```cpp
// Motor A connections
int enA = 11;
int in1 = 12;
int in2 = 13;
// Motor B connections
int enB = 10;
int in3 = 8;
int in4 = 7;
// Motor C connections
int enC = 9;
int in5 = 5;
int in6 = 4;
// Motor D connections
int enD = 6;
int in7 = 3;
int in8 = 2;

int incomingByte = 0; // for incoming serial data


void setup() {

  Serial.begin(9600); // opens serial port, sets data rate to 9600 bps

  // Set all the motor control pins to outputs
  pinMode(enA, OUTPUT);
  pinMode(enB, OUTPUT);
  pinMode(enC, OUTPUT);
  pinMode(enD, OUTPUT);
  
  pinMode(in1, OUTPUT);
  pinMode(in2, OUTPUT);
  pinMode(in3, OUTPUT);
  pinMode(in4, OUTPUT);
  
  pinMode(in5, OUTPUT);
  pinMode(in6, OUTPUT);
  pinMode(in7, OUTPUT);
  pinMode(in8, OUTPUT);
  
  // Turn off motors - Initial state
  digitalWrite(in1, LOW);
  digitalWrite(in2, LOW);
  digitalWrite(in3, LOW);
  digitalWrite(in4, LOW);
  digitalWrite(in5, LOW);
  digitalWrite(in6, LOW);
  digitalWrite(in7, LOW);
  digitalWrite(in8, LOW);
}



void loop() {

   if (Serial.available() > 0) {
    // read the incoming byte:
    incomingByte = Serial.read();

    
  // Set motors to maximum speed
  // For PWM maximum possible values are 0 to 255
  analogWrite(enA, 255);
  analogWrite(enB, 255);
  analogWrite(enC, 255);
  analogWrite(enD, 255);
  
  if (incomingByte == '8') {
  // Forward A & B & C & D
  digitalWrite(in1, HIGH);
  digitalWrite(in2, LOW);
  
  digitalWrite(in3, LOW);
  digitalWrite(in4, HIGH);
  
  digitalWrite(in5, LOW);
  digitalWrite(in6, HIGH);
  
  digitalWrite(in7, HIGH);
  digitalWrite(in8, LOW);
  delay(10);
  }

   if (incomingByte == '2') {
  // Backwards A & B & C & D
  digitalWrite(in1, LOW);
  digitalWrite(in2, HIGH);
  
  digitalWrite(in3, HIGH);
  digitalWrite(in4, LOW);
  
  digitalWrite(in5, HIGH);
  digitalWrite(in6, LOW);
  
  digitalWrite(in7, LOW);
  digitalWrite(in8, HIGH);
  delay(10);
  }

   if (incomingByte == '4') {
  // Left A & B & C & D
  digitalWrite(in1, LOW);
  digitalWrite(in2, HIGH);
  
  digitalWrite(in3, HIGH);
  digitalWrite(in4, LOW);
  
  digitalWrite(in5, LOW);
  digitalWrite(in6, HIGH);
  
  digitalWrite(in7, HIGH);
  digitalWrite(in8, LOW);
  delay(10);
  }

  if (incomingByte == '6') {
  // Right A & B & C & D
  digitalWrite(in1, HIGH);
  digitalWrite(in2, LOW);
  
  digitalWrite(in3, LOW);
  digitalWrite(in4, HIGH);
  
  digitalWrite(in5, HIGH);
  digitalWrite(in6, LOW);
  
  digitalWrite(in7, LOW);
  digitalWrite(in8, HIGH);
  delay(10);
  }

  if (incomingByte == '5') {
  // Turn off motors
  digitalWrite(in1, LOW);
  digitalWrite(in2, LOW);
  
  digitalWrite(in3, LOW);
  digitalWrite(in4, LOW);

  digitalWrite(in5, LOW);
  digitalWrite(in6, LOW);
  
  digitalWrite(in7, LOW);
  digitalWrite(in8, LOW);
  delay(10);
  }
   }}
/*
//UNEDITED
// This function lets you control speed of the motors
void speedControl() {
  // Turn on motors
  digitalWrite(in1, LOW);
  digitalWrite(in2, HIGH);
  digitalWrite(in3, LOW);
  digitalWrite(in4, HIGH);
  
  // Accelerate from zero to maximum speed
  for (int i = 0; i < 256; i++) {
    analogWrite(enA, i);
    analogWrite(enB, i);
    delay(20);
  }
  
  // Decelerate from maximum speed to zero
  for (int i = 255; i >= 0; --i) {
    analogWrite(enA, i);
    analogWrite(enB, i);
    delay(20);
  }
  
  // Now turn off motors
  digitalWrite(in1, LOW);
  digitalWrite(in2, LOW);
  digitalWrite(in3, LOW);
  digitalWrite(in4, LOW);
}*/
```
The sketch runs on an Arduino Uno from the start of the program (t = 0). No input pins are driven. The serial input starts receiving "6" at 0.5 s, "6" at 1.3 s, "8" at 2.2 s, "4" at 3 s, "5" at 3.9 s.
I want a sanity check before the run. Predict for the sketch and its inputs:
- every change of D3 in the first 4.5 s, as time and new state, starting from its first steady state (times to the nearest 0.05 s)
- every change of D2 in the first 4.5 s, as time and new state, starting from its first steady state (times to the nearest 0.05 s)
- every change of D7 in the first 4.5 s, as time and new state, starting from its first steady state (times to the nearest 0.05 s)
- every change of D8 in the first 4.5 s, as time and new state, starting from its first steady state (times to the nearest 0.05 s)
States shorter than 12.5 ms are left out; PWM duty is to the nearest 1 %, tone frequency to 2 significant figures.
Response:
0 s low; 2.2 s high; 3.9 s low
0 s low; 0.5 s high; 2.2 s low
0 s low; 0.5 s high; 3 s low
0 s low; 3 s high; 3.9 s low
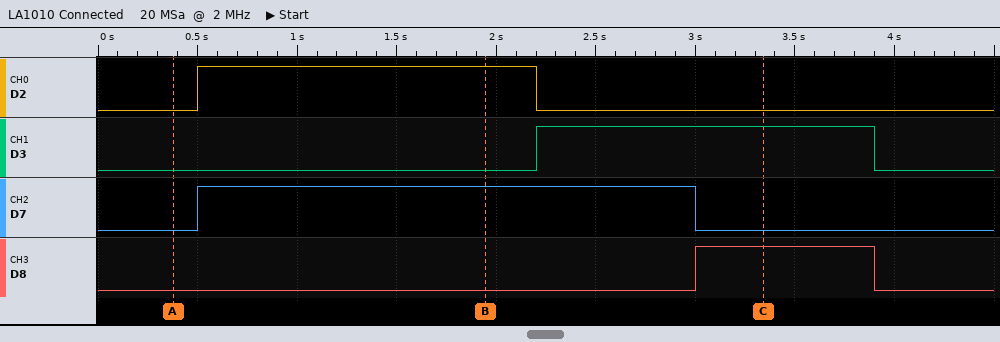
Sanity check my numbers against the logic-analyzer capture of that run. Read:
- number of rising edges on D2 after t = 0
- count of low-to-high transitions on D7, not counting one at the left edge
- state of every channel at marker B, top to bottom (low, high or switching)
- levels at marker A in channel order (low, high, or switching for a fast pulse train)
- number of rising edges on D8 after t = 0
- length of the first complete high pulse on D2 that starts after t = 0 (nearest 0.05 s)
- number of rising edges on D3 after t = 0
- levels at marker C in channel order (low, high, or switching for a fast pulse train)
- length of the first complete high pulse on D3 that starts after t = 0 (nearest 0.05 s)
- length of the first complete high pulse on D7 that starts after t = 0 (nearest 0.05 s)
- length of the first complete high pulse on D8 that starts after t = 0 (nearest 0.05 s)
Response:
1
1
D2 high, D3 low, D7 high, D8 low
D2 low, D3 low, D7 low, D8 low
1
1.70 s
1
D2 low, D3 high, D7 low, D8 high
1.70 s
2.50 s
0.90 s
